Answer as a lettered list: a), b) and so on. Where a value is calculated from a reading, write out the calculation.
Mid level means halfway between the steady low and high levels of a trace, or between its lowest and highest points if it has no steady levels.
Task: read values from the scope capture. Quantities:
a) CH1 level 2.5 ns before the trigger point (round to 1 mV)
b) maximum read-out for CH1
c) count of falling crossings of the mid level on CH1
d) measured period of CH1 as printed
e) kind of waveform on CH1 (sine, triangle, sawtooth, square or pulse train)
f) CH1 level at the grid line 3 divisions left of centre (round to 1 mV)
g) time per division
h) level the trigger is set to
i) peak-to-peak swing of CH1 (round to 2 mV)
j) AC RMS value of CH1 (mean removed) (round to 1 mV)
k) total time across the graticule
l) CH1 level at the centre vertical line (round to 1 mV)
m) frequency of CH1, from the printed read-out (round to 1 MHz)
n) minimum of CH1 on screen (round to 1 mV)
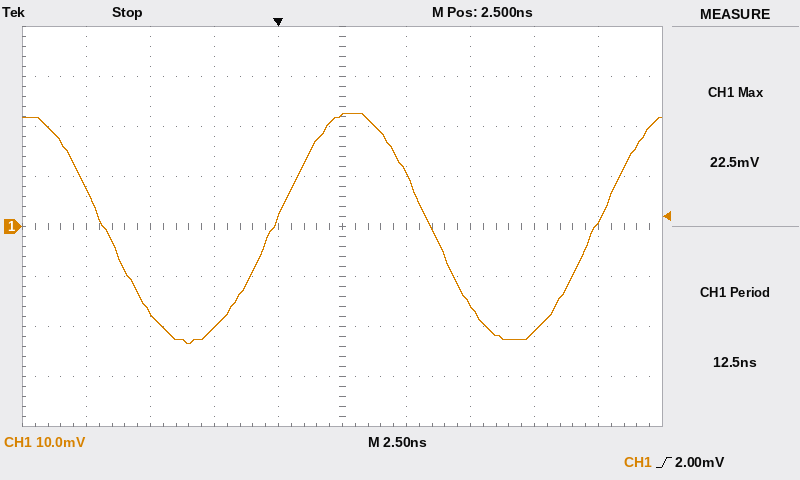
a) -20 mV
b) 22.5 mV
c) 2
d) 12.5 ns
e) sine
f) -17 mV
g) 2.5 ns
h) 2.00 mV
i) 46 mV
j) 46 mV / (2√2) ≈ 16 mV
k) 25 ns
l) 22 mV
m) 1 / 12.5 ns ≈ 80 MHz
n) -23 mV
